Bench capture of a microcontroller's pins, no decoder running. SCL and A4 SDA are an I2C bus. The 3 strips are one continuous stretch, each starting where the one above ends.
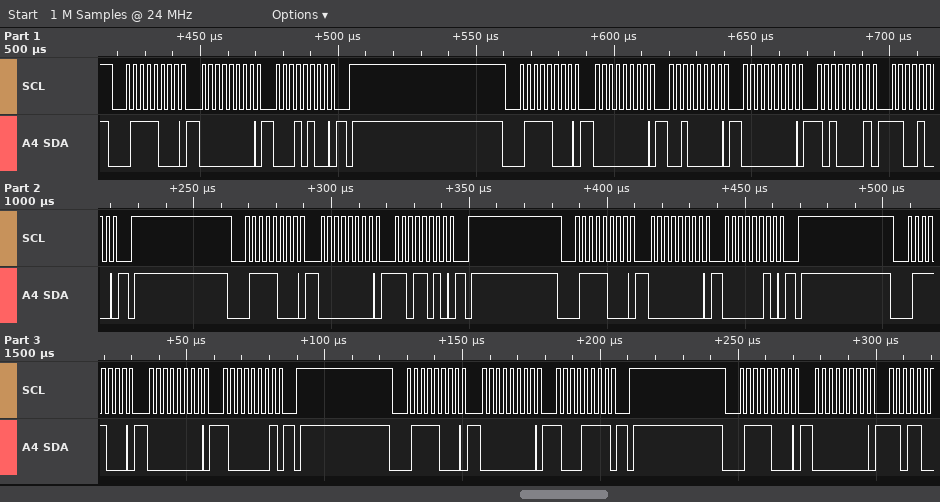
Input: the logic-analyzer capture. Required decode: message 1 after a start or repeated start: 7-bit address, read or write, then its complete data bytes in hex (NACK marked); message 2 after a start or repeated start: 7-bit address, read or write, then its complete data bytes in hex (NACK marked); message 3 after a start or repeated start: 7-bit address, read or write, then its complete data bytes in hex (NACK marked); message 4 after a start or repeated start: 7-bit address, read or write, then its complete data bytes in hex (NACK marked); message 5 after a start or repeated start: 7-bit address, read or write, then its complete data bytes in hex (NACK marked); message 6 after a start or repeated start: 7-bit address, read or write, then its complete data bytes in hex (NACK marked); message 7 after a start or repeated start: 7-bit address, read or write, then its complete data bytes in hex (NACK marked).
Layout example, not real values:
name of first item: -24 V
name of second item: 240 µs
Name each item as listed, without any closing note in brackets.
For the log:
message 1 after a start or repeated start: 7-bit address, read or write, then its complete data bytes in hex: 0x3C write: 00 14
message 2 after a start or repeated start: 7-bit address, read or write, then its complete data bytes in hex: 0x3C write: 00 20 00 A1 C8
message 3 after a start or repeated start: 7-bit address, read or write, then its complete data bytes in hex: 0x3C write: 00 DA
message 4 after a start or repeated start: 7-bit address, read or write, then its complete data bytes in hex: 0x3C write: 00 02
message 5 after a start or repeated start: 7-bit address, read or write, then its complete data bytes in hex: 0x3C write: 00 81
message 6 after a start or repeated start: 7-bit address, read or write, then its complete data bytes in hex: 0x3C write: 00 8F
message 7 after a start or repeated start: 7-bit address, read or write, then its complete data bytes in hex: 0x3C write: 00
